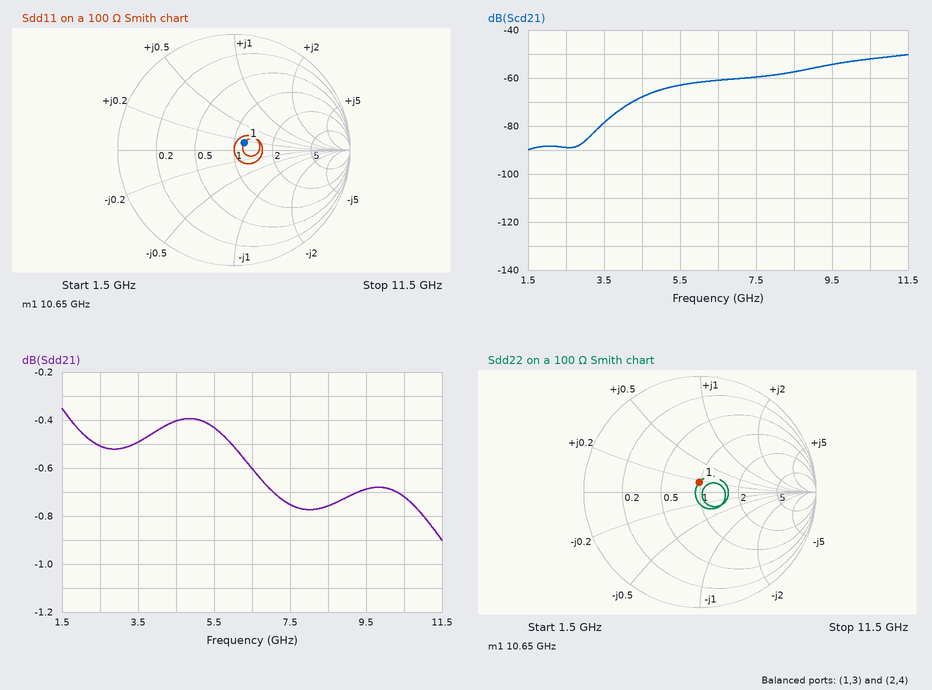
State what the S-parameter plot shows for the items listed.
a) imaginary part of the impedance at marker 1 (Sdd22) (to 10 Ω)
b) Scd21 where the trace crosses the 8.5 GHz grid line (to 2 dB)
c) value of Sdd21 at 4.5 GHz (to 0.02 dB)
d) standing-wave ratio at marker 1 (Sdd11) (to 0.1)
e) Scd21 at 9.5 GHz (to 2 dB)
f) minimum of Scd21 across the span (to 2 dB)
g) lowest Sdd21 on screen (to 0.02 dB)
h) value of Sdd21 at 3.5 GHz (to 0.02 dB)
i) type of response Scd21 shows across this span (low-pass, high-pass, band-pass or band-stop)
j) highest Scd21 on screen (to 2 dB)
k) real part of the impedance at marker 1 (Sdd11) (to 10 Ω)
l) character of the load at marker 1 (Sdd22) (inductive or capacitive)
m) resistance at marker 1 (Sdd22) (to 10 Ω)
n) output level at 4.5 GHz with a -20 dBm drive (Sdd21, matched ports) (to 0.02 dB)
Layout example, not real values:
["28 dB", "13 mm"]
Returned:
["+20 Ω", "-58 dB", "-0.40 dB", "1.2", "-54 dB", "-90 dB", "-0.90 dB", "-0.50 dB", "high-pass", "-50 dB", "120 Ω", "inductive", "100 Ω", "-20.40 dBm"]
